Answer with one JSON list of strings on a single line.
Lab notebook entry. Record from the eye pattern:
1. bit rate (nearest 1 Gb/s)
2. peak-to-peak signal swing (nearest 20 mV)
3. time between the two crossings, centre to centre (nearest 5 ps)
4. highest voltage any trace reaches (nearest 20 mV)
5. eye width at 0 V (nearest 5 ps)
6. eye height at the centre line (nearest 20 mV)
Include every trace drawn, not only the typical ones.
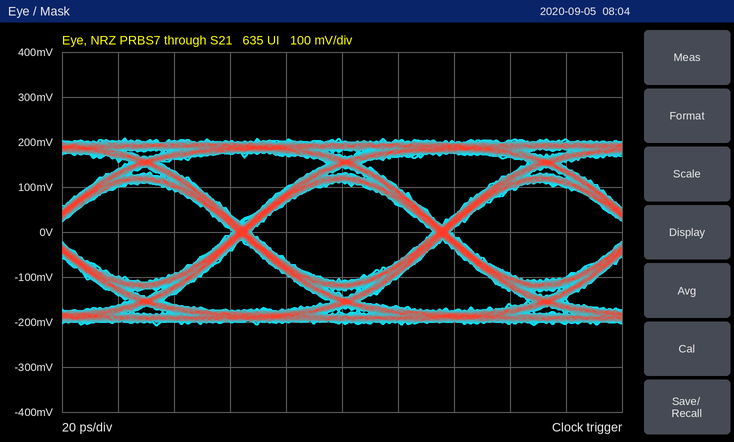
["14 Gb/s", "420 mV", "70 ps", "200 mV", "65 ps", "220 mV"]
